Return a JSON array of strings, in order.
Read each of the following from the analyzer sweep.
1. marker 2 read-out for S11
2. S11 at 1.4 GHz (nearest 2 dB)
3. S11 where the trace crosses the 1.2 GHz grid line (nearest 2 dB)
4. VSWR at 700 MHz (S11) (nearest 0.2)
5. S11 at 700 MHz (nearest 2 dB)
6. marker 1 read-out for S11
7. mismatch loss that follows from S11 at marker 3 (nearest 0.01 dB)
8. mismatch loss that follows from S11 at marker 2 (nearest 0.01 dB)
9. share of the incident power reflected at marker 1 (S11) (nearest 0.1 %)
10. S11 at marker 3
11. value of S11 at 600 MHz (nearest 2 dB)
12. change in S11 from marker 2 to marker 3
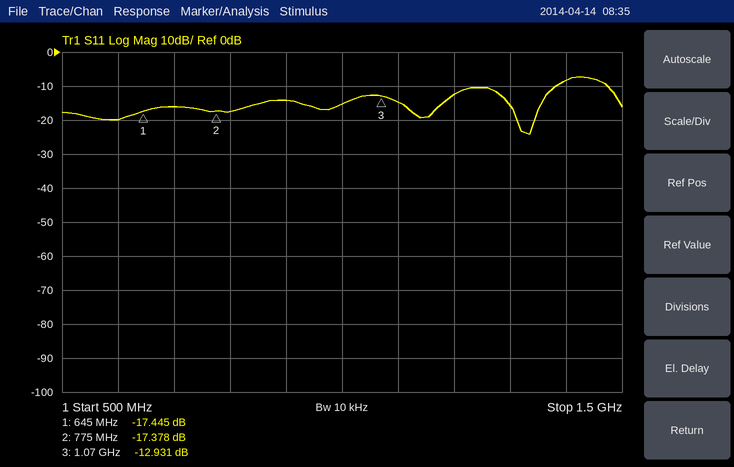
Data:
["-17.378 dB", "-8 dB", "-12 dB", "1.4", "-16 dB", "-17.445 dB", "0.23 dB", "0.08 dB", "1.8 %", "-12.931 dB", "-20 dB", "4.447 dB"]
